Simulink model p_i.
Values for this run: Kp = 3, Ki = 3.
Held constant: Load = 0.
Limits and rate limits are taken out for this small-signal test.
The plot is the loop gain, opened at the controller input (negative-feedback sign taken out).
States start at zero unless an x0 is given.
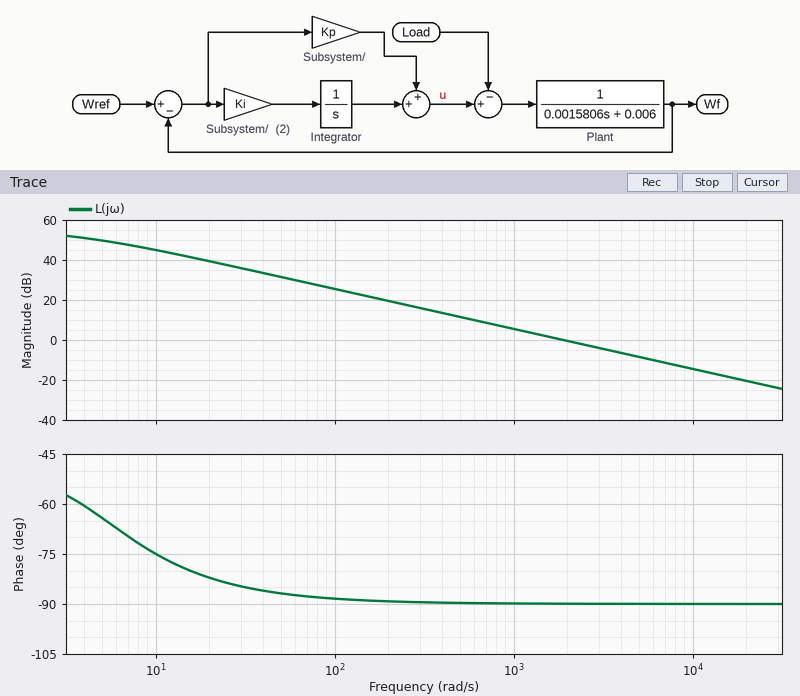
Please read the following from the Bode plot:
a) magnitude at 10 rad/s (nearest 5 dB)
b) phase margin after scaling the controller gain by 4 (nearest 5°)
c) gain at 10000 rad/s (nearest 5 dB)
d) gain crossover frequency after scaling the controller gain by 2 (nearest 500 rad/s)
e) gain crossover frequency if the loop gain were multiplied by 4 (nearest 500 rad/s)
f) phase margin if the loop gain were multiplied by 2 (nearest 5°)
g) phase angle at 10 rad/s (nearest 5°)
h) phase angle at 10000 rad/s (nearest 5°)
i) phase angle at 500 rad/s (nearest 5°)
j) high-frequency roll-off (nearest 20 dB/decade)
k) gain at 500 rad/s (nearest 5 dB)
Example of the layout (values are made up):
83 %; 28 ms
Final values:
45 dB; 90°; -15 dB; 4000 rad/s; 7500 rad/s; 90°; -75°; -90°; -90°; -20 dB/decade; 10 dB
